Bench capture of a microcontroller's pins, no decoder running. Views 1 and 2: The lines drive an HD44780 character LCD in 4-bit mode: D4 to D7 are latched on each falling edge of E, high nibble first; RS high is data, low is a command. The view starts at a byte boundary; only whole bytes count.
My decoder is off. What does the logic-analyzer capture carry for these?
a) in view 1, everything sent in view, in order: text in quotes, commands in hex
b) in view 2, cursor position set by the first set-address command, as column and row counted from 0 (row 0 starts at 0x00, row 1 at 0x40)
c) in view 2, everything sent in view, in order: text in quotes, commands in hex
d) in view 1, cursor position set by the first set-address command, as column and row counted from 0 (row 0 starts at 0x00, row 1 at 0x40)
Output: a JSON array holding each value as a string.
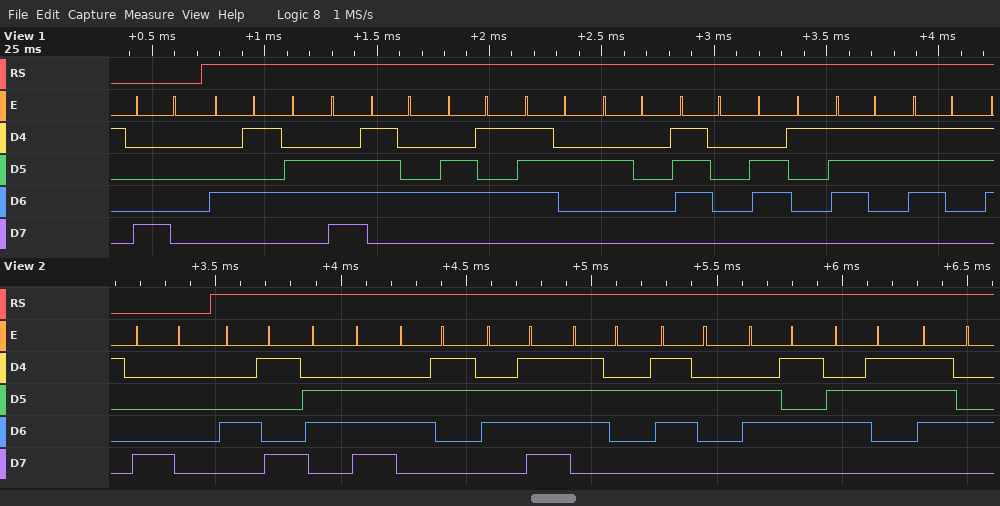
["0x80 \"Enter pass\"", "column 0, row 0", "0x80 \"Incorrect\"", "column 0, row 0"]
